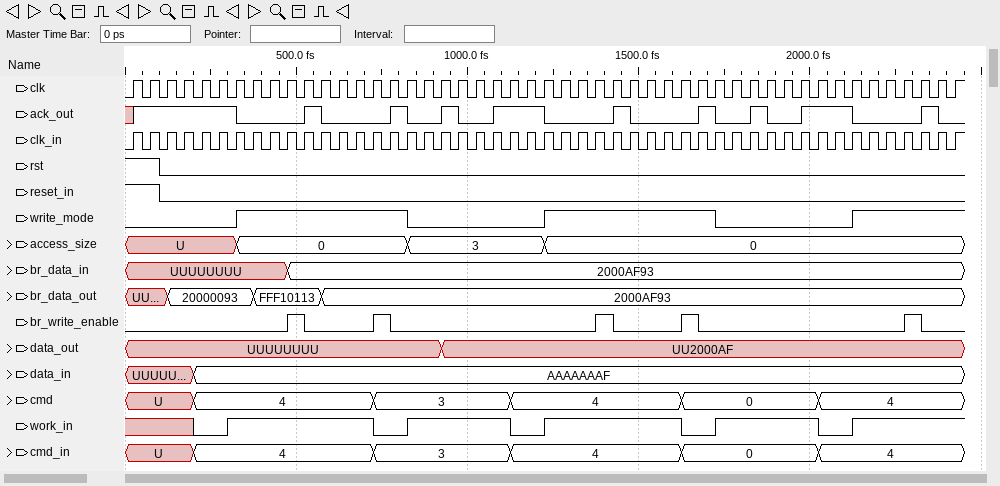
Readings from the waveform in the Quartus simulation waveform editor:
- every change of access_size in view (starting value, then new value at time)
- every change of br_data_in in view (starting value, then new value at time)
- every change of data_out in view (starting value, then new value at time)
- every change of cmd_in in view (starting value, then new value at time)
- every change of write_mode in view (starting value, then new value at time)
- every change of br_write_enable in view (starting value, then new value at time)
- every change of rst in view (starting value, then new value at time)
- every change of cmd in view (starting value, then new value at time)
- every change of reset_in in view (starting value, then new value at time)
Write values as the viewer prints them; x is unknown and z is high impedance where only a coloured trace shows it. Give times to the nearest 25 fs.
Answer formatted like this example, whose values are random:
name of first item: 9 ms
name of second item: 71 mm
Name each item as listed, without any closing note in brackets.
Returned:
every change of access_size in view: U, 0 at 325 fs, 3 at 825 fs, 0 at 1225 fs
every change of br_data_in in view: UUUUUUUU, 2000AF93 at 475 fs
every change of data_out in view: UUUUUUUU, UU2000AF at 925 fs
every change of cmd_in in view: U, 4 at 200 fs, 3 at 725 fs, 4 at 1125 fs, 0 at 1625 fs, 4 at 2025 fs
every change of write_mode in view: 0, 1 at 325 fs, 0 at 825 fs, 1 at 1225 fs, 0 at 1725 fs, 1 at 2125 fs
every change of br_write_enable in view: 0, 1 at 475 fs, 0 at 525 fs, 1 at 725 fs, 0 at 775 fs, 1 at 1375 fs, 0 at 1425 fs, 1 at 1625 fs, 0 at 1675 fs, 1 at 2275 fs, 0 at 2325 fs
every change of rst in view: 1, 0 at 100 fs
every change of cmd in view: U, 4 at 200 fs, 3 at 725 fs, 4 at 1125 fs, 0 at 1625 fs, 4 at 2025 fs
every change of reset_in in view: 1, 0 at 100 fs
